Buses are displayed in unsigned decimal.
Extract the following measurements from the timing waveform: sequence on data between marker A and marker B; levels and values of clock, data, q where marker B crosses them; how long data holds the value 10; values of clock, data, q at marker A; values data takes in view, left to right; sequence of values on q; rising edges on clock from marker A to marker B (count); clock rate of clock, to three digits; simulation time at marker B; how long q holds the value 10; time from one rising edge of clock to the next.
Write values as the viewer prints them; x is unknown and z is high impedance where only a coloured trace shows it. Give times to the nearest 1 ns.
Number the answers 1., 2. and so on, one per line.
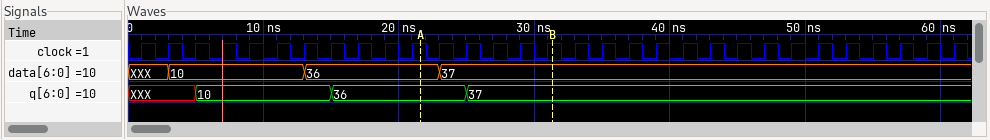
1. 36, 37
2. clock=1, data=37, q=37
3. 10 ns
4. clock=1, data=36, q=36
5. XXX, 10, 36, 37
6. XXX, 10, 36, 37
7. 5
8. 500 MHz
9. 31 ns
10. 10 ns
11. 2 ns
